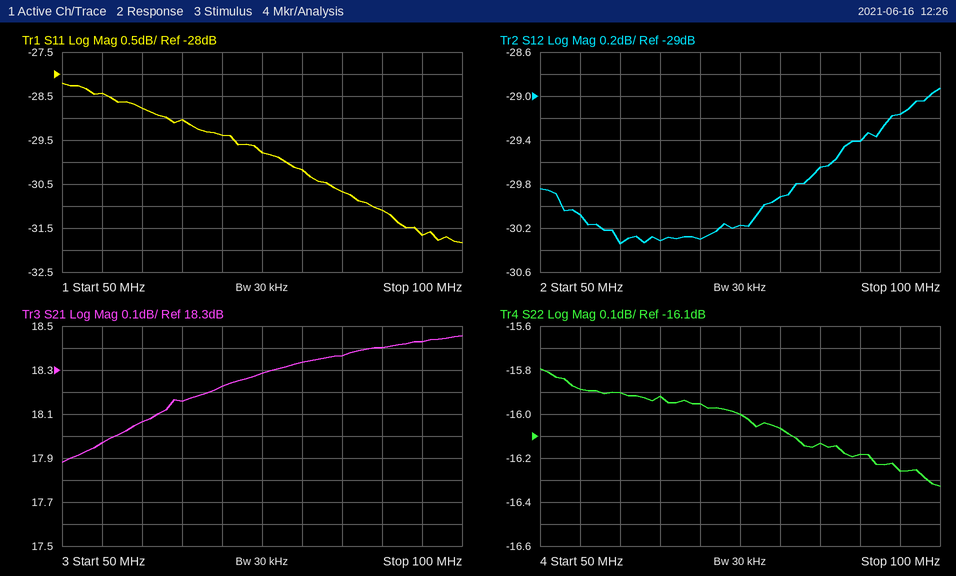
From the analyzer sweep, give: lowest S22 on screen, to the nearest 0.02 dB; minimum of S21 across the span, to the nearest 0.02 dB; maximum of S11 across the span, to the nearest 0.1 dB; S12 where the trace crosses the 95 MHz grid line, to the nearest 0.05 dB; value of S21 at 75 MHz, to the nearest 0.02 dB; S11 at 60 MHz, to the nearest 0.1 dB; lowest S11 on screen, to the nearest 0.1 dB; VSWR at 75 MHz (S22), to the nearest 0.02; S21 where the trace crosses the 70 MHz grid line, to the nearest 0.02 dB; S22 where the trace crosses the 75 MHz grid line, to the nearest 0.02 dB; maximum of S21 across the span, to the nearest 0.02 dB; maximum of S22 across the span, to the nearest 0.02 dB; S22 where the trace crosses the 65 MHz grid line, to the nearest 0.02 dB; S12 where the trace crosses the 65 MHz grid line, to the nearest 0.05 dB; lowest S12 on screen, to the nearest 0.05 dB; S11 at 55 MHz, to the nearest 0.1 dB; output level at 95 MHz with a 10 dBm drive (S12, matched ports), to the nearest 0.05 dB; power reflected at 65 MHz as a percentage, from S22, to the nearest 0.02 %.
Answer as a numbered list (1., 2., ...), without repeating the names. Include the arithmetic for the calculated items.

1. -16.32 dB
2. 17.88 dB
3. -28.2 dB
4. -29.15 dB
5. 18.28 dB
6. -28.8 dB
7. -31.8 dB
8. |Γ| = 10^(-16/20) = 0.1585; VSWR = (1 + 0.1585)/(1 − 0.1585) ≈ 1.38
9. 18.22 dB
10. -16.00 dB
11. 18.46 dB
12. -15.80 dB
13. -15.92 dB
14. -30.30 dB
15. -30.35 dB
16. -28.4 dB
17. 10 dBm + (-29.15 dB) = -19.15 dBm
18. 10^(-15.92/10) ≈ 2.56 %
